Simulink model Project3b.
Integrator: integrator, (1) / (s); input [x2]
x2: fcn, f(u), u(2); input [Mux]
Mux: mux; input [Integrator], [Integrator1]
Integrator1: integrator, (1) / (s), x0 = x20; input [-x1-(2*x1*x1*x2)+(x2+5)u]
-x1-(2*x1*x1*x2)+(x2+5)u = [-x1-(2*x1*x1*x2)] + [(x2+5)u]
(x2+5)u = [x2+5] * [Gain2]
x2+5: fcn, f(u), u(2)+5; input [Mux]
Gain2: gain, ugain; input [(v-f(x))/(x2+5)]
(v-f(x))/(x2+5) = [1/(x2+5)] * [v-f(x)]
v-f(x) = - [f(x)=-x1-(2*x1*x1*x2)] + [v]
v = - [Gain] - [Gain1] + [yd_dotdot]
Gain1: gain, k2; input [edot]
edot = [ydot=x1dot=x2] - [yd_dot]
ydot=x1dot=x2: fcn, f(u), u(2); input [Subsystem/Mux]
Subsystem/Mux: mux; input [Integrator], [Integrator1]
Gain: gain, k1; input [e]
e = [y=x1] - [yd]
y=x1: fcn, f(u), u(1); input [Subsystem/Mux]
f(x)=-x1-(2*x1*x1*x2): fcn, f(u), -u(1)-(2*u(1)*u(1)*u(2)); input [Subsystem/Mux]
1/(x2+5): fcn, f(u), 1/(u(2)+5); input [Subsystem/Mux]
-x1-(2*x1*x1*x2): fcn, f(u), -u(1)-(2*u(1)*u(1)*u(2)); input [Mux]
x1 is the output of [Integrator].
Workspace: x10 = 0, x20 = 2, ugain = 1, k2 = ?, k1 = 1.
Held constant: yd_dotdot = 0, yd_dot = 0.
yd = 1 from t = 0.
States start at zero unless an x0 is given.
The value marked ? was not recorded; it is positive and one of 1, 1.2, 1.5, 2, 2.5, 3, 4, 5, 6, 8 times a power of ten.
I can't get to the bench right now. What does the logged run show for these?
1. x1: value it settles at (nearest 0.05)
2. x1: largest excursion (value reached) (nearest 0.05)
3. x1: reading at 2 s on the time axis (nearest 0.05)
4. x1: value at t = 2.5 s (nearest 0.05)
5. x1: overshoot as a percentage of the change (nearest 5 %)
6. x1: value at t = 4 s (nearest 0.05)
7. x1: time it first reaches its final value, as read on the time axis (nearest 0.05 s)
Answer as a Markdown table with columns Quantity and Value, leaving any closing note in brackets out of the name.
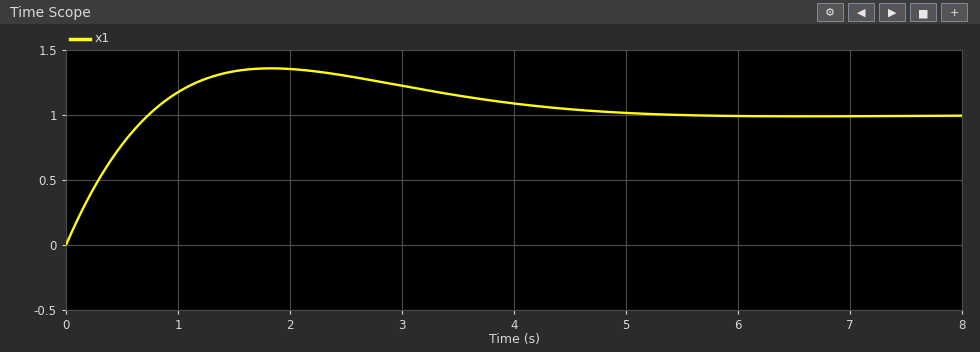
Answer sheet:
| Quantity | Value |
|---|---|
| x1: value it settles at | 1.00 |
| x1: largest excursion (value reached) | 1.35 |
| x1: reading at 2 s on the time axis | 1.35 |
| x1: value at t = 2.5 s | 1.30 |
| x1: overshoot as a percentage of the change | 35 % |
| x1: value at t = 4 s | 1.10 |
| x1: time it first reaches its final value, as read on the time axis | 0.75 s |
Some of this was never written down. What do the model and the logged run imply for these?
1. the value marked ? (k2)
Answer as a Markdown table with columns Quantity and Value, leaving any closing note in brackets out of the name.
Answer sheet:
| Quantity | Value |
|---|---|
| the value marked ? | 1.5 |
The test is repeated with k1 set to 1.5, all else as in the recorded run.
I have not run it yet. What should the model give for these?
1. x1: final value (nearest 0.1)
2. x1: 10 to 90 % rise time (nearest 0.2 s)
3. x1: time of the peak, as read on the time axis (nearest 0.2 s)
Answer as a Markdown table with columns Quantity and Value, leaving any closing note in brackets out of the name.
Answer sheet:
| Quantity | Value |
|---|---|
| x1: final value | 1.0 |
| x1: 10 to 90 % rise time | 0.6 s |
| x1: time of the peak, as read on the time axis | 1.6 s |
